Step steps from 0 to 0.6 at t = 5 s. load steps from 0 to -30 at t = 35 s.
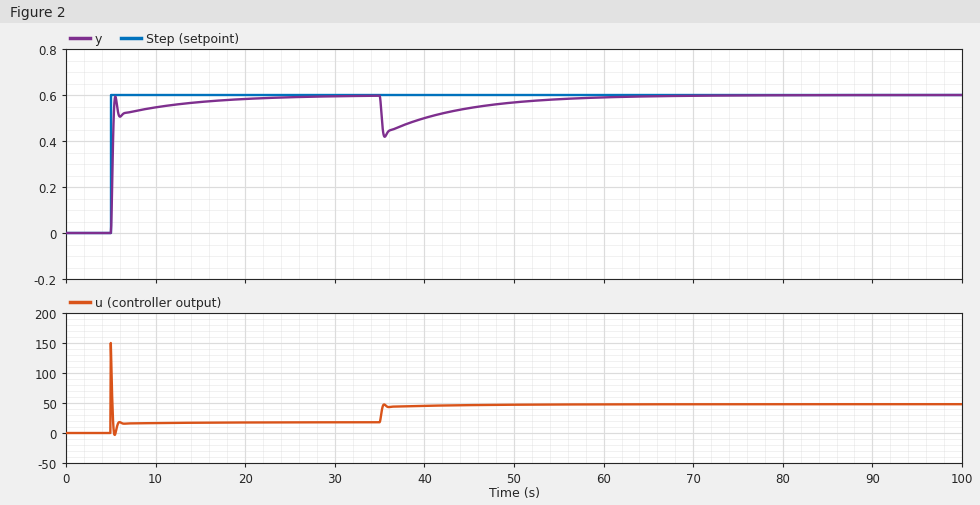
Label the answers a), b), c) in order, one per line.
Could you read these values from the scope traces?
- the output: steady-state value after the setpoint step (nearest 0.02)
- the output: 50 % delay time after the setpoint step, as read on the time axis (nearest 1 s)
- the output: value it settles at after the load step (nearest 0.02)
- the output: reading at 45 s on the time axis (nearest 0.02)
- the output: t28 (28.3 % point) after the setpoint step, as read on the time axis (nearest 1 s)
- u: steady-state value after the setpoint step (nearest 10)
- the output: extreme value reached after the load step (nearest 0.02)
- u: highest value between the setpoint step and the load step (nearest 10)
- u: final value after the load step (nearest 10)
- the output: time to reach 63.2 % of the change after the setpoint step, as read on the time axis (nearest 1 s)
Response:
a) 0.60
b) 5 s
c) 0.60
d) 0.54
e) 5 s
f) 20
g) 0.42
h) 150
i) 50
j) 5 s
